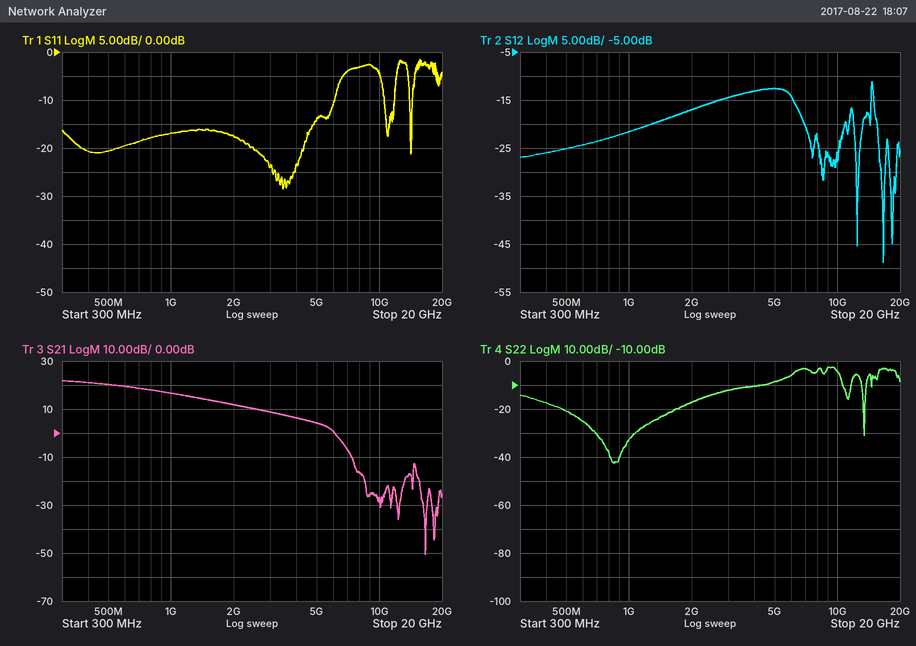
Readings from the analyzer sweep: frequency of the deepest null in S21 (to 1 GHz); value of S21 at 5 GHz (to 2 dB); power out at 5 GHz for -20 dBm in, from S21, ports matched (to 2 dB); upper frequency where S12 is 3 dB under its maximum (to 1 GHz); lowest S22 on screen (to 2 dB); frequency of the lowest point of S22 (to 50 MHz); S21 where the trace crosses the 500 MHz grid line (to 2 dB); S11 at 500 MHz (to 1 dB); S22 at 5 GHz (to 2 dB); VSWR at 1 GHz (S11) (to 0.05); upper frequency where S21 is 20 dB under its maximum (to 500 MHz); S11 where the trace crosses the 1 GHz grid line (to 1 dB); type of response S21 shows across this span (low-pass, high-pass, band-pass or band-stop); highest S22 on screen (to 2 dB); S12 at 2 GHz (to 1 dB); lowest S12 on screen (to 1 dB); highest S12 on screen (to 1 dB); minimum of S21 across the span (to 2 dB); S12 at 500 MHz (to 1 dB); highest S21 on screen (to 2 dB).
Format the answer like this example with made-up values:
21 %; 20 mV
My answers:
17 GHz; 4 dB; -16 dBm; 15 GHz; -42 dB; 850 MHz; 20 dB; -21 dB; -8 dB; 1.35; 6.0 GHz; -17 dB; low-pass; -2 dB; -17 dB; -49 dB; -11 dB; -50 dB; -25 dB; 22 dB
